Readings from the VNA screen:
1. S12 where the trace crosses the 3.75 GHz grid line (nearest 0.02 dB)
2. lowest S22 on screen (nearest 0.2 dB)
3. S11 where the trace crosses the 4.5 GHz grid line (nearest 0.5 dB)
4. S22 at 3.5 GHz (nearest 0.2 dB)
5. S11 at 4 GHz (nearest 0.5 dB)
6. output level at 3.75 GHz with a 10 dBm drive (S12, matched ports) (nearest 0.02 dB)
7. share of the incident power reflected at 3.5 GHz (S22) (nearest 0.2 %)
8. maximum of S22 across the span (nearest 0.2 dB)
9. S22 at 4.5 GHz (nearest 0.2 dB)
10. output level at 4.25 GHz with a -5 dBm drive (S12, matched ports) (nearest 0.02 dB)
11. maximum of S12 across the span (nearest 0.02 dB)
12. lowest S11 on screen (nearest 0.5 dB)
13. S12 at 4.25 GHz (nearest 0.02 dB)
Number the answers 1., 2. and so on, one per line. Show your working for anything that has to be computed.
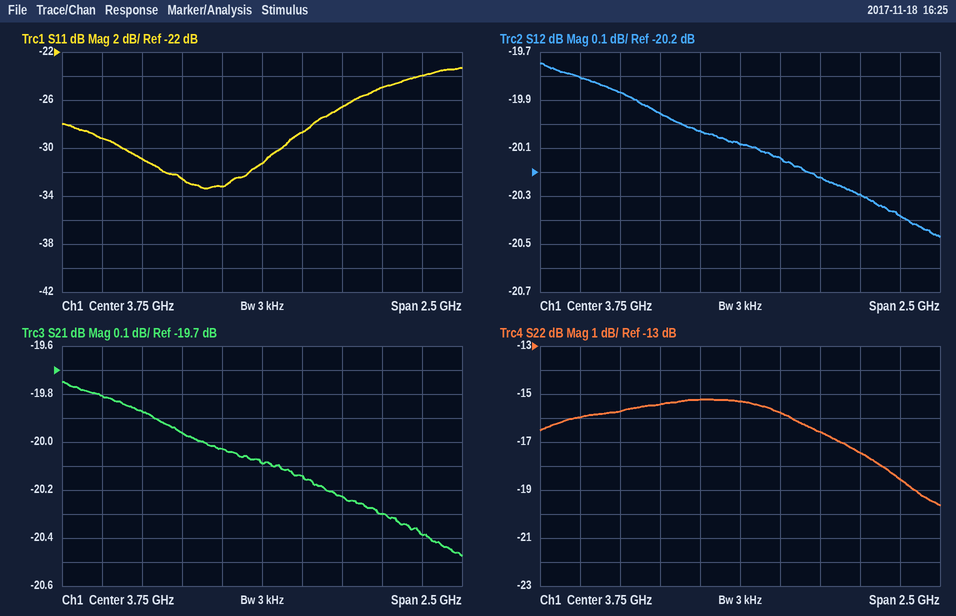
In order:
1. -20.08 dB
2. -19.6 dB
3. -25.0 dB
4. -15.2 dB
5. -28.5 dB
6. 10 dBm + (-20.08 dB) = -10.08 dBm
7. 10^(-15.2/10) ≈ 3.0 %
8. -15.2 dB
9. -17.4 dB
10. -5 dBm + (-20.22 dB) = -25.22 dBm
11. -19.74 dB
12. -33.5 dB
13. -20.22 dB
